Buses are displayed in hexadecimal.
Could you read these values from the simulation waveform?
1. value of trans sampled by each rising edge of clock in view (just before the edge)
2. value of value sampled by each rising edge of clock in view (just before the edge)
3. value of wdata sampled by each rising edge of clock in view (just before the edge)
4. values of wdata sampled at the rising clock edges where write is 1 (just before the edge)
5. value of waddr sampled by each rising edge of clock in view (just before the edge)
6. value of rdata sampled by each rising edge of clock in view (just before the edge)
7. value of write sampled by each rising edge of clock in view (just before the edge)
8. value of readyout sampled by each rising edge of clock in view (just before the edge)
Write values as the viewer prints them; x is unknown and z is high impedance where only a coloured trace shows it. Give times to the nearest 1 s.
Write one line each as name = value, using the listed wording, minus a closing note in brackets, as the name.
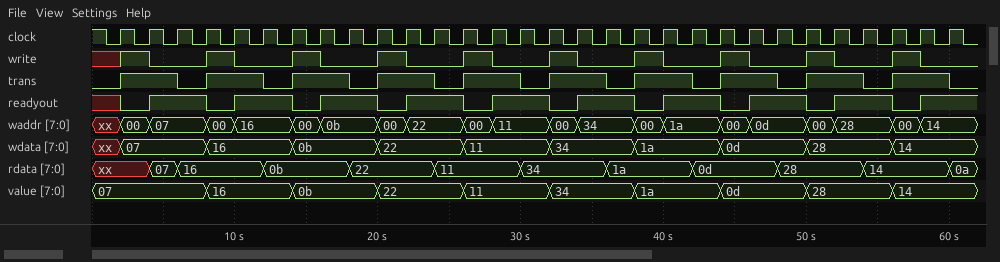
value of trans sampled by each rising edge of clock in view = 0 1 1 0 1 1 0 1 1 0 1 1 0 1 1 0 1 1 0 1 1 0 1 1 0 1 1 0 1 1
value of value sampled by each rising edge of clock in view = 07, 07, 07, 07, 16, 16, 16, 0b, 0b, 0b, 22, 22, 22, 11, 11, 11, 34, 34, 34, 1a, 1a, 1a, 0d, 0d, 0d, 28, 28, 28, 14, 14
value of wdata sampled by each rising edge of clock in view = xx, 07, 07, 07, 16, 16, 16, 0b, 0b, 0b, 22, 22, 22, 11, 11, 11, 34, 34, 34, 1a, 1a, 1a, 0d, 0d, 0d, 28, 28, 28, 14, 14
values of wdata sampled at the rising clock edges where write is 1 = 07, 16, 0b, 22, 11, 34, 1a, 0d, 28, 14
value of waddr sampled by each rising edge of clock in view = xx, 00, 07, 07, 00, 16, 16, 00, 0b, 0b, 00, 22, 22, 00, 11, 11, 00, 34, 34, 00, 1a, 1a, 00, 0d, 0d, 00, 28, 28, 00, 14
value of rdata sampled by each rising edge of clock in view = xx, xx, 07, 16, 16, 16, 0b, 0b, 0b, 22, 22, 22, 11, 11, 11, 34, 34, 34, 1a, 1a, 1a, 0d, 0d, 0d, 28, 28, 28, 14, 14, 14
value of write sampled by each rising edge of clock in view = x 1 0 0 1 0 0 1 0 0 1 0 0 1 0 0 1 0 0 1 0 0 1 0 0 1 0 0 1 0
value of readyout sampled by each rising edge of clock in view = x 0 1 1 0 1 1 0 1 1 0 1 1 0 1 1 0 1 1 0 1 1 0 1 1 0 1 1 0 1
